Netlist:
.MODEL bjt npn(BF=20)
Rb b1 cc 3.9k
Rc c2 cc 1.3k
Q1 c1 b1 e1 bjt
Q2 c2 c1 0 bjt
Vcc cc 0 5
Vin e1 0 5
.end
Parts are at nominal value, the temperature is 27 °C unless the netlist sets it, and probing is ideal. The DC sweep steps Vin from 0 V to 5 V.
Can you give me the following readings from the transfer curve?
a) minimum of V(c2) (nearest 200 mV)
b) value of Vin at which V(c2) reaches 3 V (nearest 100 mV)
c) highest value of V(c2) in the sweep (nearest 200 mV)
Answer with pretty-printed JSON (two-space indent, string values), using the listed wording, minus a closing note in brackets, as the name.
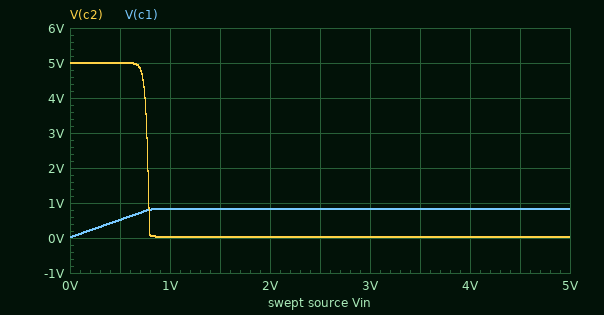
{
  "minimum of V(c2)": "0 V",
  "value of Vin at which V(c2) reaches 3 V": "800 mV",
  "highest value of V(c2) in the sweep": "5.0 V"
}
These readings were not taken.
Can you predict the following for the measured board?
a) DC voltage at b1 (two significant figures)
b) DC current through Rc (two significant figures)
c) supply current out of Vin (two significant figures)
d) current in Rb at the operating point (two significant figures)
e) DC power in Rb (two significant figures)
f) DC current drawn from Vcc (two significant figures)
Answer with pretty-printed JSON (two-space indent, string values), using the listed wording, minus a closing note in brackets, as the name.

{
  "DC voltage at b1": "1.6 V",
  "DC current through Rc": "3.8 mA",
  "supply current out of Vin": "870 µA",
  "current in Rb at the operating point": "870 µA",
  "DC power in Rb": "3.0 mW",
  "DC current drawn from Vcc": "4.7 mA"
}
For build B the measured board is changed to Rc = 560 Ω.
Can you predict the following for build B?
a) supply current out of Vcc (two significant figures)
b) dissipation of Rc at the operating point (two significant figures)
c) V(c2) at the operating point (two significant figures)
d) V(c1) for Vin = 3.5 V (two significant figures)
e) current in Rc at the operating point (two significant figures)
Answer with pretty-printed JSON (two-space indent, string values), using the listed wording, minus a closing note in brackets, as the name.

{
  "supply current out of Vcc": "9.7 mA",
  "dissipation of Rc at the operating point": "44 mW",
  "V(c2) at the operating point": "58 mV",
  "V(c1) for Vin = 3.5 V": "840 mV",
  "current in Rc at the operating point": "8.8 mA"
}
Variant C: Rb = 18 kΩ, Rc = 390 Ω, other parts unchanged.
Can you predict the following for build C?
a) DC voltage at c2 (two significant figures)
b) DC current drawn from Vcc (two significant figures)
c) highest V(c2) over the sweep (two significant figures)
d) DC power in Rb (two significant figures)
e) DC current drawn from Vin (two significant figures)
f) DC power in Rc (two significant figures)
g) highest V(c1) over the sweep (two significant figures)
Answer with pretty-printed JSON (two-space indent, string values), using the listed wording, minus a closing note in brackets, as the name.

{
  "DC voltage at c2": "2.0 V",
  "DC current drawn from Vcc": "7.8 mA",
  "highest V(c2) over the sweep": "5.0 V",
  "DC power in Rb": "660 µW",
  "DC current drawn from Vin": "190 µA",
  "DC power in Rc": "23 mW",
  "highest V(c1) over the sweep": "830 mV"
}
